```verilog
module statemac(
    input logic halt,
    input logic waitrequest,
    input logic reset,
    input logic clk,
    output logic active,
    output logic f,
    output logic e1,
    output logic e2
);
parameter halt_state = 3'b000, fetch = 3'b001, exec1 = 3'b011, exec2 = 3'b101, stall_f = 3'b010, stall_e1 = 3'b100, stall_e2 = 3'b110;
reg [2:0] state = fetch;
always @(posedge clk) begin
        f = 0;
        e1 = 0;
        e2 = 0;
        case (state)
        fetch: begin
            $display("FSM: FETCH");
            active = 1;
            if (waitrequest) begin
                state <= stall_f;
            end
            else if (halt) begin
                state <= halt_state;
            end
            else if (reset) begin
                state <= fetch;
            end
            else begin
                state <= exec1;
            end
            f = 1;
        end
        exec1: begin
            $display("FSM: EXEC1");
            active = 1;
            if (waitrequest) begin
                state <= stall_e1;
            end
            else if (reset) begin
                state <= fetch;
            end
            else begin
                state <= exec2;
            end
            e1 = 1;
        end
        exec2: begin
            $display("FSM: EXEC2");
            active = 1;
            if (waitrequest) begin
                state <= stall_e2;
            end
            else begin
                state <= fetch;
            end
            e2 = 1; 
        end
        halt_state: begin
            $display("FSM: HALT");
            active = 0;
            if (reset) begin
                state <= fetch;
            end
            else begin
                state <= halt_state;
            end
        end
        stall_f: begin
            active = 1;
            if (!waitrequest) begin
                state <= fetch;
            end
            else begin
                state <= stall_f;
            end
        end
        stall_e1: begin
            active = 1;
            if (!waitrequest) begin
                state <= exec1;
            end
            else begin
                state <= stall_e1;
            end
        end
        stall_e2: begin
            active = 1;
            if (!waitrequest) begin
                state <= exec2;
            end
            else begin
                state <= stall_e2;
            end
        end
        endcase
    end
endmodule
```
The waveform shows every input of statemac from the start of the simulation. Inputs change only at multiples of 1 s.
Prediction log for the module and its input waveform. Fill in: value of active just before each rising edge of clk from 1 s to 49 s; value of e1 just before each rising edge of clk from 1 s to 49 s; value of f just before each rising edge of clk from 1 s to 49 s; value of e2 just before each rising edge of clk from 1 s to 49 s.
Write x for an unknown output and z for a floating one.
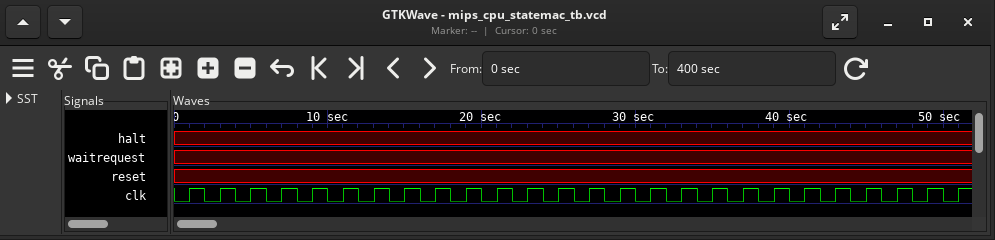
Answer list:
x 1 1 1 1 1 1 1 1 1 1 1 1 1 1 1 1 1 1 1 1 1 1 1 1
x 0 1 0 0 1 0 0 1 0 0 1 0 0 1 0 0 1 0 0 1 0 0 1 0
x 1 0 0 1 0 0 1 0 0 1 0 0 1 0 0 1 0 0 1 0 0 1 0 0
x 0 0 1 0 0 1 0 0 1 0 0 1 0 0 1 0 0 1 0 0 1 0 0 1
